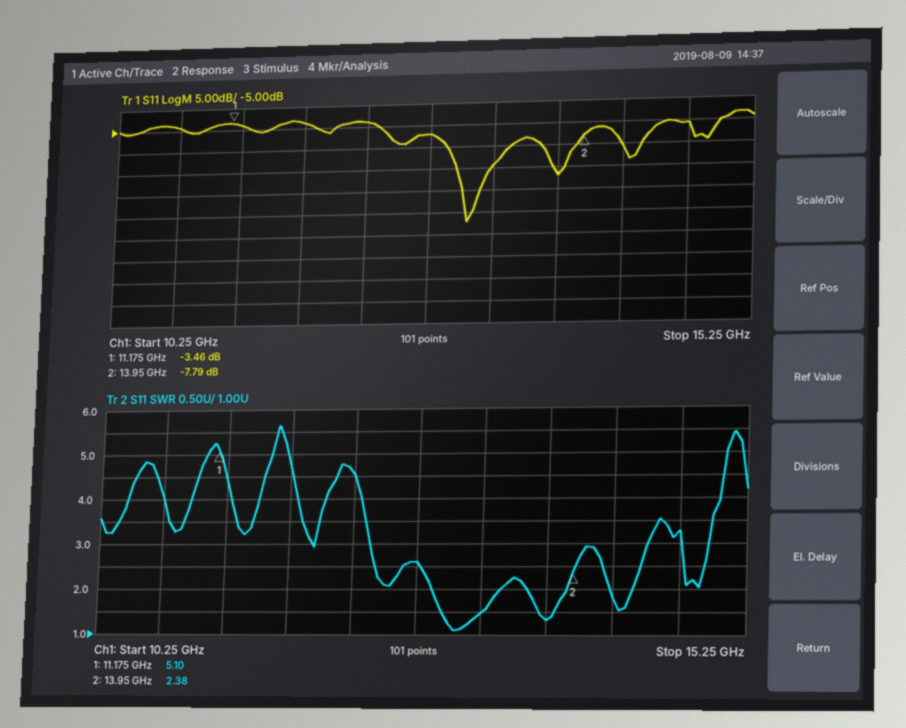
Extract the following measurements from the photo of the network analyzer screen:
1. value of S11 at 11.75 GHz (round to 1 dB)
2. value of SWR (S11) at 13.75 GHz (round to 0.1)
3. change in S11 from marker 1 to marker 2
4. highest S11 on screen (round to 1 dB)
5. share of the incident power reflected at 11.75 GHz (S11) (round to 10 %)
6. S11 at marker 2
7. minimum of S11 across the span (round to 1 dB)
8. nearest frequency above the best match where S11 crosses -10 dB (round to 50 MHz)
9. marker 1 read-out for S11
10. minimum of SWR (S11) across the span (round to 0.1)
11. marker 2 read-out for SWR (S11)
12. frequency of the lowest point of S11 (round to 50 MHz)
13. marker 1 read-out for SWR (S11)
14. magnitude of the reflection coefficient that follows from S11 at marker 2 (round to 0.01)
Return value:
-4 dB
1.3
-4.33 dB
-3 dB
40 %
-7.79 dB
-27 dB
13.40 GHz
-3.46 dB
1.1
2.38
13.05 GHz
5.10
0.41
